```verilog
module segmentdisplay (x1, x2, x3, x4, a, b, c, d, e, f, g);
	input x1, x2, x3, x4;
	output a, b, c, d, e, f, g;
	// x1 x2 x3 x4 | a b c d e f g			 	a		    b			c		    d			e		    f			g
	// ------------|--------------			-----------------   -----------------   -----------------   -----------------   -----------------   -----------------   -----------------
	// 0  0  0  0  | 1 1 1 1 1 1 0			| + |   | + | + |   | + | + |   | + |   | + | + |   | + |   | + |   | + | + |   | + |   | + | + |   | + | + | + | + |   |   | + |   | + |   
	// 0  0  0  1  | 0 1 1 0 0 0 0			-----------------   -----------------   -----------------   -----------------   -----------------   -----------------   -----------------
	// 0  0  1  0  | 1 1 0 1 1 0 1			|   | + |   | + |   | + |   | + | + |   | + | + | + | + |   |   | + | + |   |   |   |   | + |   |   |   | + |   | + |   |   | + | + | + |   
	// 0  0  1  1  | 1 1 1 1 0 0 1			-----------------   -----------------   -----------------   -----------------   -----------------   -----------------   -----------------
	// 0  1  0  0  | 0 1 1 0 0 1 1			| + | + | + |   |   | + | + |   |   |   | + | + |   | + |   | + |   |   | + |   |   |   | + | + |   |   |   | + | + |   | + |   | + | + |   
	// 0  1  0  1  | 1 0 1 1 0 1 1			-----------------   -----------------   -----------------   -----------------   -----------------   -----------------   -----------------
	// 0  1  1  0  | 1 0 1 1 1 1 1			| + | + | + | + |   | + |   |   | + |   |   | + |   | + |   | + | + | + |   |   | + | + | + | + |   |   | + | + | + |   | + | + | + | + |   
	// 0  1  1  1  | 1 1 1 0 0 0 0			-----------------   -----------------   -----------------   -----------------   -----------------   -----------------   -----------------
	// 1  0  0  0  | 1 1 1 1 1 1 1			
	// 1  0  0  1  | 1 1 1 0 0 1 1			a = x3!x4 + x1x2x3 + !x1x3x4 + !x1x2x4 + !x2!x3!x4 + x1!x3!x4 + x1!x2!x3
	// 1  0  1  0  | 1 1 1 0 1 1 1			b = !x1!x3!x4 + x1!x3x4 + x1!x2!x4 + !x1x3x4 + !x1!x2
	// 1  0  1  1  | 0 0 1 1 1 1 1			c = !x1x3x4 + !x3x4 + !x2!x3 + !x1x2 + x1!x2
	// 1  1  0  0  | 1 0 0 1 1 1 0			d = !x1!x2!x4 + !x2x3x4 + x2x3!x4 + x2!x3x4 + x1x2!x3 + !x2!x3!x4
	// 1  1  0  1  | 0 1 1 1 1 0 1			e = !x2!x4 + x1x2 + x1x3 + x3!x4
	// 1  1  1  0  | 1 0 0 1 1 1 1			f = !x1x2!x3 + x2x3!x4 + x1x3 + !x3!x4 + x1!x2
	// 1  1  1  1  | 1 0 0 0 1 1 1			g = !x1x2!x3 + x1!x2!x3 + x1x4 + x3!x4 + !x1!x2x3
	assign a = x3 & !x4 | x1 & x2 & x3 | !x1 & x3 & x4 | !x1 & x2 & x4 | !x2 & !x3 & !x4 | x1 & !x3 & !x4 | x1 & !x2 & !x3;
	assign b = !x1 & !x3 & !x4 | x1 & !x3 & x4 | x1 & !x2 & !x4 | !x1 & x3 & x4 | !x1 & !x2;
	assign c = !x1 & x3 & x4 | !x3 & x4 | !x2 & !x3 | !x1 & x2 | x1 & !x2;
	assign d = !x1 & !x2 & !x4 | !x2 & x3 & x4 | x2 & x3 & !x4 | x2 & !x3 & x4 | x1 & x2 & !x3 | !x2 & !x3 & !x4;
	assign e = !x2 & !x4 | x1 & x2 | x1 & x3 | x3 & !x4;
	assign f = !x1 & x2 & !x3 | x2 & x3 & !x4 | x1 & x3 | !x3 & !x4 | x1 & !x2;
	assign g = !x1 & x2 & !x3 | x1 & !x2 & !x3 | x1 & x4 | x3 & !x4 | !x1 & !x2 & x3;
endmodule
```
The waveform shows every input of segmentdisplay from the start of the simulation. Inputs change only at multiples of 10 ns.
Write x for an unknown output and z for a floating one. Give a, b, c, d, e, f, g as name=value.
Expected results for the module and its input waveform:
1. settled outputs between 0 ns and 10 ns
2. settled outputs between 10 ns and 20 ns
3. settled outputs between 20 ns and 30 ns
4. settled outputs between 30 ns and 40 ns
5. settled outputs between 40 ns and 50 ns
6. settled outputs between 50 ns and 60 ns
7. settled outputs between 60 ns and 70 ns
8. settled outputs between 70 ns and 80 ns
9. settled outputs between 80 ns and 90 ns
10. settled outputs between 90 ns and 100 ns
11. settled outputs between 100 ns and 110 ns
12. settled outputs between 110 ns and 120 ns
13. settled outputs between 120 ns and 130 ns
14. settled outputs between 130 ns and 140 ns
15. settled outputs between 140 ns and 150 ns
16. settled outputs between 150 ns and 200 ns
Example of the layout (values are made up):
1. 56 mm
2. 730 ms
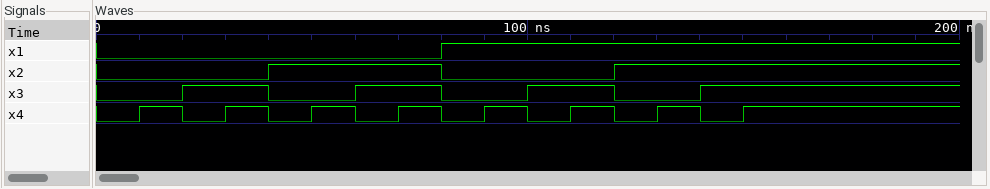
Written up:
1. a=1, b=1, c=1, d=1, e=1, f=1, g=0
2. a=0, b=1, c=1, d=0, e=0, f=0, g=0
3. a=1, b=1, c=0, d=1, e=1, f=0, g=1
4. a=1, b=1, c=1, d=1, e=0, f=0, g=1
5. a=0, b=1, c=1, d=0, e=0, f=1, g=1
6. a=1, b=0, c=1, d=1, e=0, f=1, g=1
7. a=1, b=0, c=1, d=1, e=1, f=1, g=1
8. a=1, b=1, c=1, d=0, e=0, f=0, g=0
9. a=1, b=1, c=1, d=1, e=1, f=1, g=1
10. a=1, b=1, c=1, d=0, e=0, f=1, g=1
11. a=1, b=1, c=1, d=0, e=1, f=1, g=1
12. a=0, b=0, c=1, d=1, e=1, f=1, g=1
13. a=1, b=0, c=0, d=1, e=1, f=1, g=0
14. a=0, b=1, c=1, d=1, e=1, f=0, g=1
15. a=1, b=0, c=0, d=1, e=1, f=1, g=1
16. a=1, b=0, c=0, d=0, e=1, f=1, g=1
